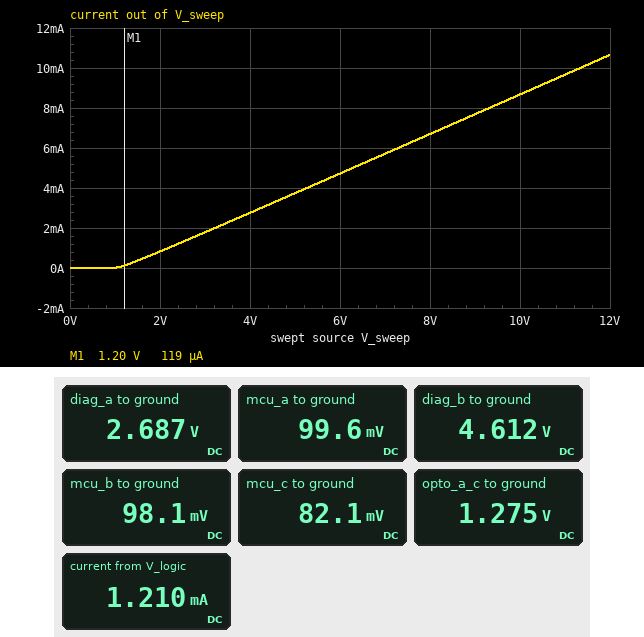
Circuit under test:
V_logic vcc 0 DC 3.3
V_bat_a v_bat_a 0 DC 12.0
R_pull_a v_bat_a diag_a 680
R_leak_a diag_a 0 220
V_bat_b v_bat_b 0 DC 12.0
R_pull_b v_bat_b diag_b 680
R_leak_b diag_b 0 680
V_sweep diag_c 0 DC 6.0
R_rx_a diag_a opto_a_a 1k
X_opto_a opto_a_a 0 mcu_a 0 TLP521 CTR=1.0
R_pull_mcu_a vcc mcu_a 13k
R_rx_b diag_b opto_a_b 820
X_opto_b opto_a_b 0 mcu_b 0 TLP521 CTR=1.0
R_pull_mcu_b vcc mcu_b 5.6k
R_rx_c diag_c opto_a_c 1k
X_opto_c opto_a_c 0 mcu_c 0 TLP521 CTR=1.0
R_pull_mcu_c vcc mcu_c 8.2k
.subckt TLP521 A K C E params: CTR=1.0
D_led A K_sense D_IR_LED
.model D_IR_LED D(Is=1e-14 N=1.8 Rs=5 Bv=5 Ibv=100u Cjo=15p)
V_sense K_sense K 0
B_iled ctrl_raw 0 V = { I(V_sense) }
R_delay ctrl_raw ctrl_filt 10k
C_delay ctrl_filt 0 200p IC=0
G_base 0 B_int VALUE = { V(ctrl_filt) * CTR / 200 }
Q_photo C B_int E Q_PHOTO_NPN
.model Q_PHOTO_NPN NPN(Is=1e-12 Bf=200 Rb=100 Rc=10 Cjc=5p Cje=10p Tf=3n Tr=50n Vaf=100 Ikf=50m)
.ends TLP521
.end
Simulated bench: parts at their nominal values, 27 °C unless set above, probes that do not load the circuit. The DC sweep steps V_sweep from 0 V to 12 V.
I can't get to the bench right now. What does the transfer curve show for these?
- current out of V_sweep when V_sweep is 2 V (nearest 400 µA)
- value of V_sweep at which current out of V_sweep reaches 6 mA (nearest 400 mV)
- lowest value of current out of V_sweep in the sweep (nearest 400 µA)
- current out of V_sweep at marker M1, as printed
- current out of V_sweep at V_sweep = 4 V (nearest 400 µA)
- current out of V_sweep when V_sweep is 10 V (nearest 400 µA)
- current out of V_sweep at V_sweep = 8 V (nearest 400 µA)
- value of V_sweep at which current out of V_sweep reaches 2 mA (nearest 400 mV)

800 µA
7.2 V
0 A
119 µA
2.8 mA
8.8 mA
6.8 mA
3.2 V
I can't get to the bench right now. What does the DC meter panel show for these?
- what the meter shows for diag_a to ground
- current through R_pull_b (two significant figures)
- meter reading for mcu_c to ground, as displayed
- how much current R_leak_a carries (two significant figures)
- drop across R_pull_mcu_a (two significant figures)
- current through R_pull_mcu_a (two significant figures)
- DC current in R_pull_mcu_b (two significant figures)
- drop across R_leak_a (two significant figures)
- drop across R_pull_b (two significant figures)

2.687 V
11 mA
82.1 mV
12 mA
3.2 V
250 µA
570 µA
2.7 V
7.4 V
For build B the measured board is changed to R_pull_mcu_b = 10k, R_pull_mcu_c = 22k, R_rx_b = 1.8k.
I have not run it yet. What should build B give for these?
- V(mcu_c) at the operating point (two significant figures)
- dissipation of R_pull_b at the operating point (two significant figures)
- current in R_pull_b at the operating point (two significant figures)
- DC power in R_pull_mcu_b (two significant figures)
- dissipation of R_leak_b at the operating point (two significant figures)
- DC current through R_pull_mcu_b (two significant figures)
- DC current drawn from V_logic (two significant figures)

57 mV
67 mW
9.9 mA
1.0 mW
40 mW
320 µA
710 µA
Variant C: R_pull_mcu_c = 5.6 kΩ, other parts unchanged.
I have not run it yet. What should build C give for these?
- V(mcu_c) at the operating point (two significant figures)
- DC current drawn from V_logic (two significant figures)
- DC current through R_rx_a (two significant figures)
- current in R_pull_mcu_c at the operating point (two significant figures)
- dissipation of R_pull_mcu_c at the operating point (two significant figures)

94 mV
1.4 mA
1.5 mA
570 µA
1.8 mW
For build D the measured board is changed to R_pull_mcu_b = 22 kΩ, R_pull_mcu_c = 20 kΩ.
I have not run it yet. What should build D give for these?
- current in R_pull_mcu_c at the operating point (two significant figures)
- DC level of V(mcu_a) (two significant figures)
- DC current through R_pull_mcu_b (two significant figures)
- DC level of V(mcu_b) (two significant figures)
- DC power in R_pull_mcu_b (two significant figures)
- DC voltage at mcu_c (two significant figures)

160 µA
100 mV
150 µA
60 mV
480 µW
59 mV
